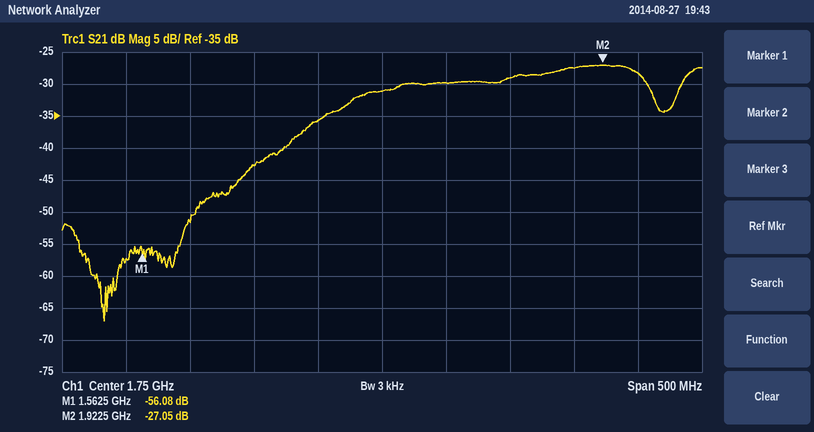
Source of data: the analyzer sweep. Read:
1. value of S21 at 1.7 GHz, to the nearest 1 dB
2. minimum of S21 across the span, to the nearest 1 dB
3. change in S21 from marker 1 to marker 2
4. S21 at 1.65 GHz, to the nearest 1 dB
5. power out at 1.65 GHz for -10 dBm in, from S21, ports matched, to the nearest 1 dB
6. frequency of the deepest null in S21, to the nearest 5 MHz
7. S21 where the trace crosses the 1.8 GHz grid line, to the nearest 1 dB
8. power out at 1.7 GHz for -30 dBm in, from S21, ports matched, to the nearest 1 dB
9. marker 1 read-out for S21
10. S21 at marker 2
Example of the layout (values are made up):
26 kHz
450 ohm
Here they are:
-36 dB
-67 dB
29.03 dB
-43 dB
-53 dBm
1.535 GHz
-30 dB
-66 dBm
-56.08 dB
-27.05 dB
